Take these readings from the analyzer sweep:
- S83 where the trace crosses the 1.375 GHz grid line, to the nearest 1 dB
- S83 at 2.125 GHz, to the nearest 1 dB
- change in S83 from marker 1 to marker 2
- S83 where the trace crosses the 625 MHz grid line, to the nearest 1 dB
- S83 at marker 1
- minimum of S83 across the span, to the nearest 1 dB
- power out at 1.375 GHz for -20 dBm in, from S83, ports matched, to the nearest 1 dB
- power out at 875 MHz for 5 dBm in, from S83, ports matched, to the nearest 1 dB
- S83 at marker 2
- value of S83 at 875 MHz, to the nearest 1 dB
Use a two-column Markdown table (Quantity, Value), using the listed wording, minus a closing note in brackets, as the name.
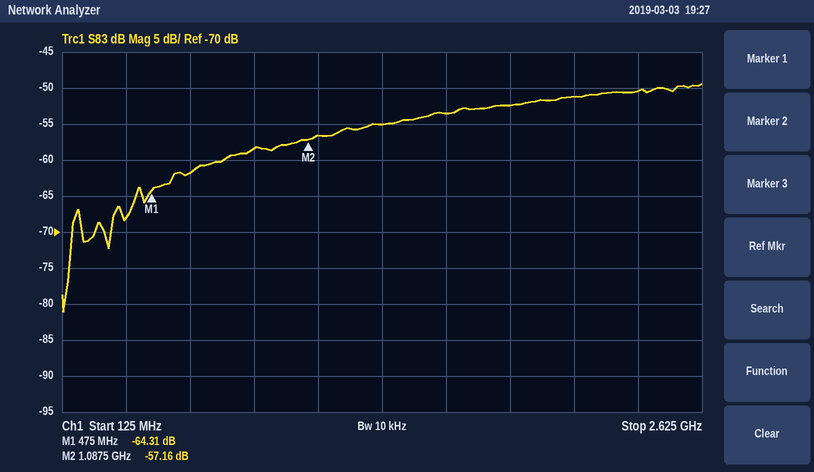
| Quantity | Value |
|---|---|
| S83 where the trace crosses the 1.375 GHz grid line, to the nearest 1 dB | -55 dB |
| S83 at 2.125 GHz, to the nearest 1 dB | -51 dB |
| change in S83 from marker 1 to marker 2 | 7.15 dB |
| S83 where the trace crosses the 625 MHz grid line, to the nearest 1 dB | -62 dB |
| S83 at marker 1 | -64.31 dB |
| minimum of S83 across the span, to the nearest 1 dB | -81 dB |
| power out at 1.375 GHz for -20 dBm in, from S83, ports matched, to the nearest 1 dB | -75 dBm |
| power out at 875 MHz for 5 dBm in, from S83, ports matched, to the nearest 1 dB | -53 dBm |
| S83 at marker 2 | -57.16 dB |
| value of S83 at 875 MHz, to the nearest 1 dB | -58 dB |
